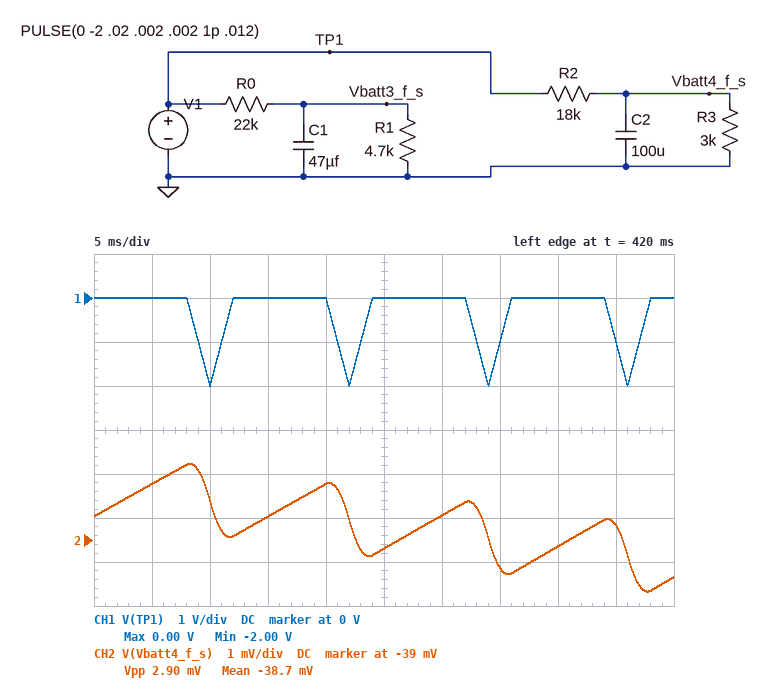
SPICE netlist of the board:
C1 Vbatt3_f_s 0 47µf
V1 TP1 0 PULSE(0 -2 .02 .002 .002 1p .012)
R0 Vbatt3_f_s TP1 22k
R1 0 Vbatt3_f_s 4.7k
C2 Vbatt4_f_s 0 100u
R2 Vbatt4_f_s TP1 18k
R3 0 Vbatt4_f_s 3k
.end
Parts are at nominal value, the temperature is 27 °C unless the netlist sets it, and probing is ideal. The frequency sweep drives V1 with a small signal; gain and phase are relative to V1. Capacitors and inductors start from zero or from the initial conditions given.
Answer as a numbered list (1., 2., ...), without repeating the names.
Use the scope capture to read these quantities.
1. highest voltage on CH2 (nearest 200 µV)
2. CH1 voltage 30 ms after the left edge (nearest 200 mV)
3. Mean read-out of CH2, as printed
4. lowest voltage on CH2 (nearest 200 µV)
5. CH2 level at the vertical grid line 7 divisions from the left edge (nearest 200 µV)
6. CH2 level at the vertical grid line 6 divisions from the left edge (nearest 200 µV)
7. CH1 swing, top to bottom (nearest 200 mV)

1. -37.2 mV
2. 0 V
3. -38.7 mV
4. -40.2 mV
5. -39.6 mV
6. -38.4 mV
7. 2.0 V
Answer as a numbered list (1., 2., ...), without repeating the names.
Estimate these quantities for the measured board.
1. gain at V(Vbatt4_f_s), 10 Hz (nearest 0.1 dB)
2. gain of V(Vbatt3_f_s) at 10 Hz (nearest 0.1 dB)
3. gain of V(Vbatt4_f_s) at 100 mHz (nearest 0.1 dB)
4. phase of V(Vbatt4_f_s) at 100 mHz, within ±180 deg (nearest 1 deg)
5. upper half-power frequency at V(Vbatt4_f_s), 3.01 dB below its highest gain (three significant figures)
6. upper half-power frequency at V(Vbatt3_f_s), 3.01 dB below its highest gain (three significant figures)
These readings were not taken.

1. -41.1 dB
2. -36.3 dB
3. -17.0 dB
4. -9 deg
5. 619 mHz
6. 874 mHz
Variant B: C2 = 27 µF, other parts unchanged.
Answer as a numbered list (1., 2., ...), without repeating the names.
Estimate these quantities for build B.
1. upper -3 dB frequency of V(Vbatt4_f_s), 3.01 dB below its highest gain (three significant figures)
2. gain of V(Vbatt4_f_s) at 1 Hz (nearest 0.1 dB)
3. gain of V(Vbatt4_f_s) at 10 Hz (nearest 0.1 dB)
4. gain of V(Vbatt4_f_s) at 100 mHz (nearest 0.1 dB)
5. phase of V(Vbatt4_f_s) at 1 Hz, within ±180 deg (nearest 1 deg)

1. 2.29 Hz
2. -17.7 dB
3. -29.9 dB
4. -16.9 dB
5. -24 deg
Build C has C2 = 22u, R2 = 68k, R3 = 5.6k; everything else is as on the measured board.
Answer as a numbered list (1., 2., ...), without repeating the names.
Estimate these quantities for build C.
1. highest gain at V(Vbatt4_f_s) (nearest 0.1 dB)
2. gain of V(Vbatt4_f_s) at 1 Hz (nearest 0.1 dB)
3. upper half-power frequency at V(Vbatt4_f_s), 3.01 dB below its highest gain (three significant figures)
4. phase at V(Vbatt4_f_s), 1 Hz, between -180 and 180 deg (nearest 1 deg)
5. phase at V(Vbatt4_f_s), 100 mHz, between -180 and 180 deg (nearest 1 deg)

1. -22.4 dB
2. -24.2 dB
3. 1.40 Hz
4. -36 deg
5. -4 deg
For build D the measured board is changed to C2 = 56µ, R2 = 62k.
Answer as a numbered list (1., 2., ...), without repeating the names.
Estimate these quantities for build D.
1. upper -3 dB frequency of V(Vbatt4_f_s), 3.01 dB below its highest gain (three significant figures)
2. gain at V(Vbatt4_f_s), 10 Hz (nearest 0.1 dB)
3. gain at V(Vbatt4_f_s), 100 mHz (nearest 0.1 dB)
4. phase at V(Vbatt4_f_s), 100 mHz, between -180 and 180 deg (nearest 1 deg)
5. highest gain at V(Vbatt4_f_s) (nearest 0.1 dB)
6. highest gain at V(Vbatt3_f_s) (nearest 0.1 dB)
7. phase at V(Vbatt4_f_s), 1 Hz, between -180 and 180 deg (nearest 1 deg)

1. 993 mHz
2. -46.8 dB
3. -26.8 dB
4. -6 deg
5. -26.7 dB
6. -15.1 dB
7. -45 deg
